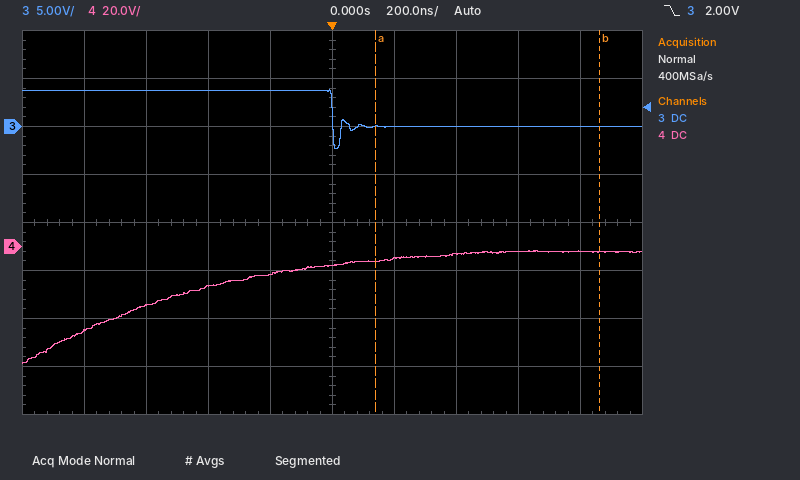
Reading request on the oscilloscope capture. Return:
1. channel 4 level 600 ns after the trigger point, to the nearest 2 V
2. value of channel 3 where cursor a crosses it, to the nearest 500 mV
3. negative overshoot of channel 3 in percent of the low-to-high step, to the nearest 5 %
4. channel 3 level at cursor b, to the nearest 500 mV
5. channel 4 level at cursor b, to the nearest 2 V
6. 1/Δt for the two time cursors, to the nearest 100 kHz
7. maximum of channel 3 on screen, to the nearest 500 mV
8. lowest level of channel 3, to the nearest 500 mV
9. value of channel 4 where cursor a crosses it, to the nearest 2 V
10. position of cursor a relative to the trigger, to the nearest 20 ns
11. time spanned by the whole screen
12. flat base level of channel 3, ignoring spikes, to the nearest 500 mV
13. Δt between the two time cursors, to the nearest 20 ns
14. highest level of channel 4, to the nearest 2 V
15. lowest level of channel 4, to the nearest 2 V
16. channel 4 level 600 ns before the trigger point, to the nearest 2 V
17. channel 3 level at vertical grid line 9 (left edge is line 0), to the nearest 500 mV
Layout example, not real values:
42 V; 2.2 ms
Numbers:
-2 V; 0.0 V; 60 %; 0.0 V; -2 V; 1.4 MHz; 4.0 V; -2.5 V; -6 V; +140 ns; 2 µs; 0.0 V; 720 ns; -2 V; -48 V; -24 V; 0.0 V
